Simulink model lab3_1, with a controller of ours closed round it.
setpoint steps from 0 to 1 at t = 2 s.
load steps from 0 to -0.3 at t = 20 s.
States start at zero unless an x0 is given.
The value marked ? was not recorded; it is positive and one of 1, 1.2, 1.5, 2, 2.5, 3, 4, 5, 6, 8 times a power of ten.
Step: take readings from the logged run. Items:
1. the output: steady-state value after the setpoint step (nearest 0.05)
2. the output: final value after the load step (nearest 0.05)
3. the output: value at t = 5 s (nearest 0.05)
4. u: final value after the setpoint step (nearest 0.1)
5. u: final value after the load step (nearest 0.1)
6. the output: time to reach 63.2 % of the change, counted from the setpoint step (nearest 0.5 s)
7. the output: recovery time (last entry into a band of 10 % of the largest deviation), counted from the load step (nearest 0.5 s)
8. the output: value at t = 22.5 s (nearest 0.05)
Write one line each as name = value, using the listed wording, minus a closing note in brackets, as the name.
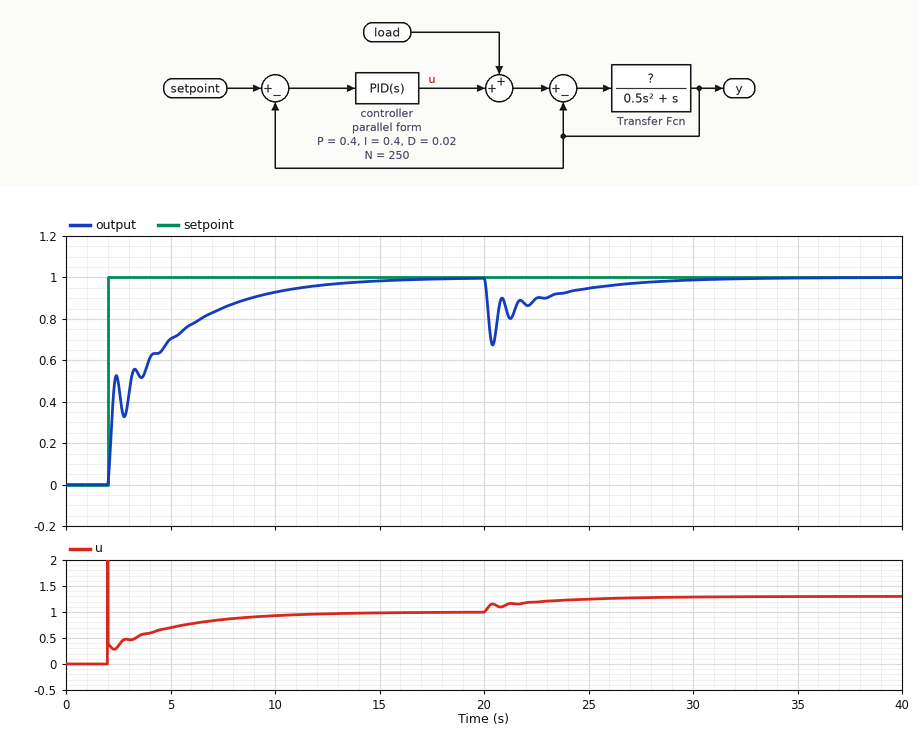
the output: steady-state value after the setpoint step = 1.00
the output: final value after the load step = 1.00
the output: value at t = 5 s = 0.70
u: final value after the setpoint step = 1.0
u: final value after the load step = 1.3
the output: time to reach 63.2 % of the change, counted from the setpoint step = 2.0 s
the output: recovery time (last entry into a band of 10 % of the largest deviation), counted from the load step = 6.5 s
the output: value at t = 22.5 s = 0.90
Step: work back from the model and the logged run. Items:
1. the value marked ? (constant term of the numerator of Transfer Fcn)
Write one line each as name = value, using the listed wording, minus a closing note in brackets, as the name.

the value marked ? = 20
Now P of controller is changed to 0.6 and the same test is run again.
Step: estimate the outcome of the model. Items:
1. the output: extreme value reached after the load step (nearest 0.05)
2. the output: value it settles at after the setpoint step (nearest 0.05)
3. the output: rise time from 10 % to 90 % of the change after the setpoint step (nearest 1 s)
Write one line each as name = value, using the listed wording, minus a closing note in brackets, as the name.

the output: extreme value reached after the load step = 0.70
the output: value it settles at after the setpoint step = 1.00
the output: rise time from 10 % to 90 % of the change after the setpoint step = 7 s
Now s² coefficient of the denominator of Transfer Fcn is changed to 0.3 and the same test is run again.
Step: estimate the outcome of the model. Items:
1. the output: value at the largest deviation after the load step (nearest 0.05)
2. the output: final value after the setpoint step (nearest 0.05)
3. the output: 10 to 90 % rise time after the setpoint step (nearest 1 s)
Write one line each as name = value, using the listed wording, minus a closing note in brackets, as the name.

the output: value at the largest deviation after the load step = 0.70
the output: final value after the setpoint step = 1.00
the output: 10 to 90 % rise time after the setpoint step = 7 s
